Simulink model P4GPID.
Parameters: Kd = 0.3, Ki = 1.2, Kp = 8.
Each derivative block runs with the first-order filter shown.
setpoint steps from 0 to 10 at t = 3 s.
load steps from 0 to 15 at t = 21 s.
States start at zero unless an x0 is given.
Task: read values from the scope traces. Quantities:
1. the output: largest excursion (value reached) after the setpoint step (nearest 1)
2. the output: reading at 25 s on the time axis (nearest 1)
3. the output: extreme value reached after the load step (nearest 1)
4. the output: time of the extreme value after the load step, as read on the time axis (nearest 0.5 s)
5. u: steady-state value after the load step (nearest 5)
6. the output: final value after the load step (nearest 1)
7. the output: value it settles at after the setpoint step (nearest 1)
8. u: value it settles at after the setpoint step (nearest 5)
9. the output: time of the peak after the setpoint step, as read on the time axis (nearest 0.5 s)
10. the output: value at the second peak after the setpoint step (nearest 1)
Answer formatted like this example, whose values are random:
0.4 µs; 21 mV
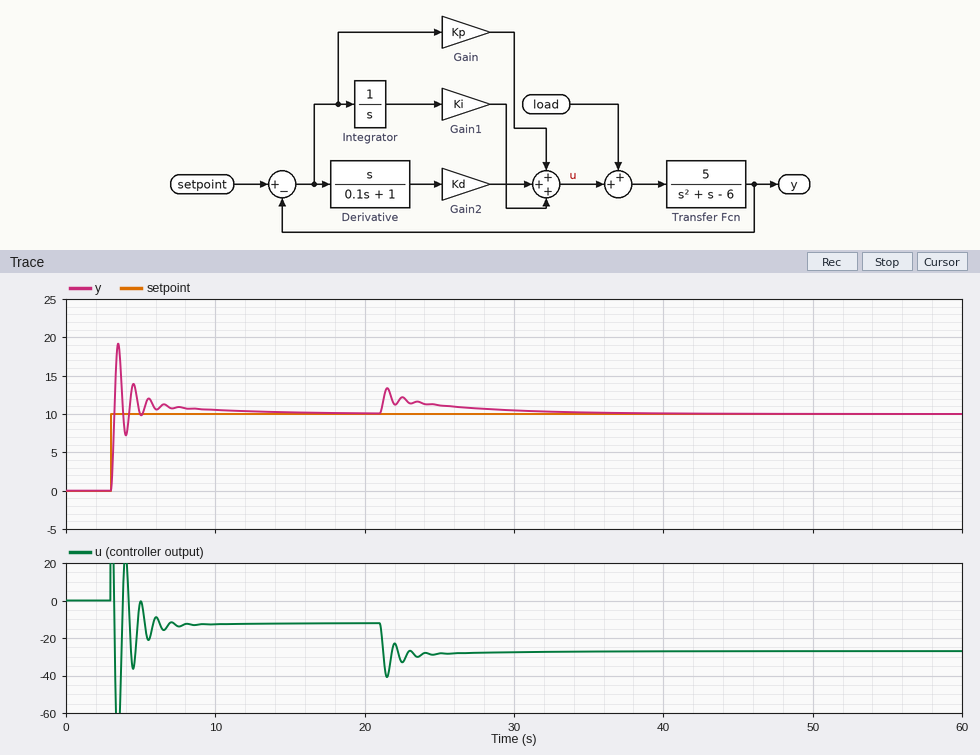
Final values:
19; 11; 13; 21.5 s; -25; 10; 10; -10; 3.5 s; 14
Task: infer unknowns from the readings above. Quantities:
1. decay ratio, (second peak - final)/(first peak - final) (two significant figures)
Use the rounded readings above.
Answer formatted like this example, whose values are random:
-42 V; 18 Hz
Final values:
0.44
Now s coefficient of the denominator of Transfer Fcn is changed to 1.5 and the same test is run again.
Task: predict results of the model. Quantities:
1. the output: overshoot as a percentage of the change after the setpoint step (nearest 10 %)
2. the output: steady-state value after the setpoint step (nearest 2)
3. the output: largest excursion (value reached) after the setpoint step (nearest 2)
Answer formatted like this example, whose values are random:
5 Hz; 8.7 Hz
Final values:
80 %; 10; 18
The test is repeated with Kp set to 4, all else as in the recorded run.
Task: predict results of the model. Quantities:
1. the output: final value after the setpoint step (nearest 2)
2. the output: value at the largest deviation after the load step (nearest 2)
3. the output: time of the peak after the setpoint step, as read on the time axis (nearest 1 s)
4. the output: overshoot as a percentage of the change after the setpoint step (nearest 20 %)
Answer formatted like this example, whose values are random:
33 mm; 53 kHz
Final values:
10; 16; 4 s; 100 %
